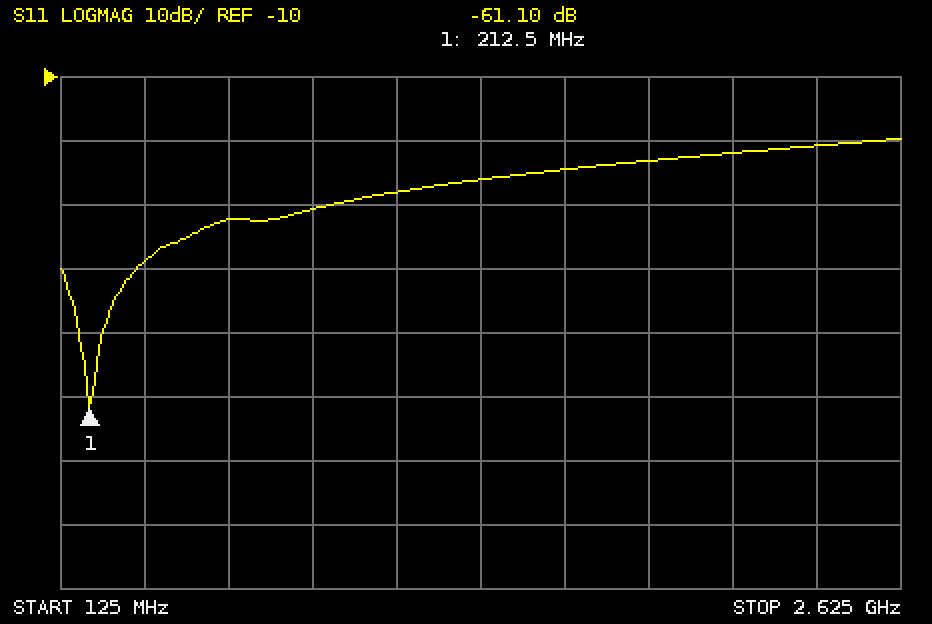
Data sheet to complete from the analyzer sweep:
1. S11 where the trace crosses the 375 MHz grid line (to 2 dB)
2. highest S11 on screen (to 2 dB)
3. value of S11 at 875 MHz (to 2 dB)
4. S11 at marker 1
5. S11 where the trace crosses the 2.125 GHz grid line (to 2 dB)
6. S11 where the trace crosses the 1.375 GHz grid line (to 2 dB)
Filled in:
-38 dB
-20 dB
-30 dB
-61.10 dB
-22 dB
-26 dB
